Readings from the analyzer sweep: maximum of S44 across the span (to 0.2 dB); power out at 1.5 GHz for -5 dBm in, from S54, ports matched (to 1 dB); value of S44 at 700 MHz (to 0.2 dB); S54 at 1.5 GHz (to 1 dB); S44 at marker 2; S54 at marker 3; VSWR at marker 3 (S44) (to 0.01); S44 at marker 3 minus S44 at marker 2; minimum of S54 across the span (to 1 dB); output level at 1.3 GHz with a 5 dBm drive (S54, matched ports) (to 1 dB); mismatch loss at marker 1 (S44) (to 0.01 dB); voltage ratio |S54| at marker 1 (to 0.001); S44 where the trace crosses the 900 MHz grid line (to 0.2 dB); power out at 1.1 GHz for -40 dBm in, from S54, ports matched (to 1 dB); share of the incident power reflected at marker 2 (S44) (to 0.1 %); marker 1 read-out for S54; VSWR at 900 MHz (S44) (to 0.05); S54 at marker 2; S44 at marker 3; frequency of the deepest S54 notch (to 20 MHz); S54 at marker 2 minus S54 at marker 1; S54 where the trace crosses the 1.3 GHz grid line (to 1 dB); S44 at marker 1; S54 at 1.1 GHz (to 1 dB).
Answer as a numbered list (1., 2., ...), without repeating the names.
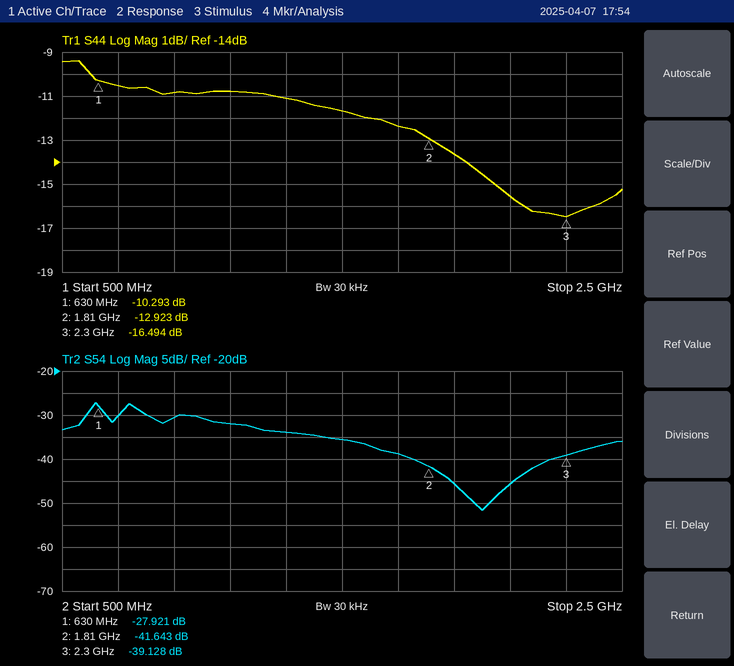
1. -9.4 dB
2. -41 dBm
3. -10.6 dB
4. -36 dB
5. -12.923 dB
6. -39.128 dB
7. 1.35
8. -3.571 dB
9. -52 dB
10. -29 dBm
11. 0.43 dB
12. 0.040
13. -10.8 dB
14. -72 dBm
15. 5.1 %
16. -27.921 dB
17. 1.80
18. -41.643 dB
19. -16.494 dB
20. 2.00 GHz
21. -13.722 dB
22. -34 dB
23. -10.293 dB
24. -32 dB
